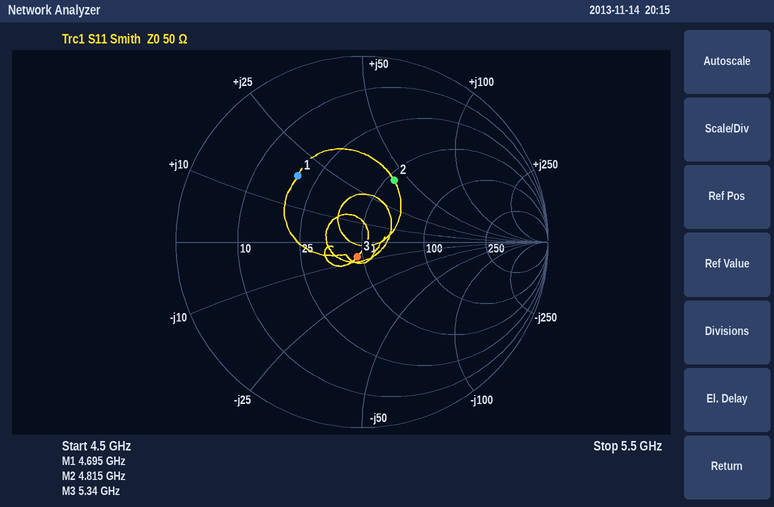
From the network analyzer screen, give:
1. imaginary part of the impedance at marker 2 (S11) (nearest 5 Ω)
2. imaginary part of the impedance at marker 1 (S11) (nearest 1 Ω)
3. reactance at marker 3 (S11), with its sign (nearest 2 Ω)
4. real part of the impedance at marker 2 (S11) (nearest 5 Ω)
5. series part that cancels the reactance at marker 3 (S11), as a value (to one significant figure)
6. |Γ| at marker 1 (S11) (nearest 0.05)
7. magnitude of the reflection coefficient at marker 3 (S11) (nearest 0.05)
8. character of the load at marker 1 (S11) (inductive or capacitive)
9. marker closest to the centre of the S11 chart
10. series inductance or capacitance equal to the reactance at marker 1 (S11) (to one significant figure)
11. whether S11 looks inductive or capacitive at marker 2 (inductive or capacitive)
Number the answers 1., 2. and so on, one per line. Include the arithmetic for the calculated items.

1. +40 Ω
2. +18 Ω
3. -8 Ω
4. 55 Ω
5. L = 8 Ω/(2π × 5.34 GHz) ≈ 238 pH, so 200 pH to one significant figure
6. 0.50
7. 0.10
8. inductive
9. marker 3
10. L = 18 Ω/(2π × 4.695 GHz) ≈ 610 pH, so 600 pH to one significant figure
11. inductive
